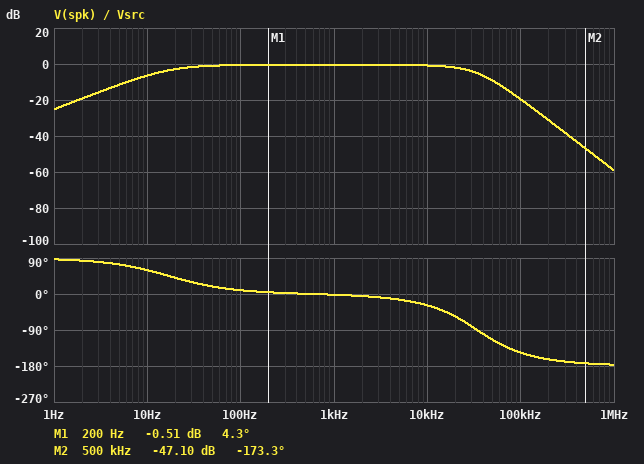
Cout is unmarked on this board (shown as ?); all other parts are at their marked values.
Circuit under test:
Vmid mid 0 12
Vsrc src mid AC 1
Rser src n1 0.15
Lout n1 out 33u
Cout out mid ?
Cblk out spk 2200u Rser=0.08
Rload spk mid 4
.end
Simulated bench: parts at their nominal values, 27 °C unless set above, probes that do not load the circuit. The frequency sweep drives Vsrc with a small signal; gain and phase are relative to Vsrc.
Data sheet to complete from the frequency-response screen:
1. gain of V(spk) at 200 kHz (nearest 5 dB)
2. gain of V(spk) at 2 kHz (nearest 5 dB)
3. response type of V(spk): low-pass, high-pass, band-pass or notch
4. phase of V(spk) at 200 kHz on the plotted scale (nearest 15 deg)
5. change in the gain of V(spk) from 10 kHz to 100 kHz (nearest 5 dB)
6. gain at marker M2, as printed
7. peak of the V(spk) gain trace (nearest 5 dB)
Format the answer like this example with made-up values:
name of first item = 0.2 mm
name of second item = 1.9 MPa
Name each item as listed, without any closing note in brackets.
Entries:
gain of V(spk) at 200 kHz = -30 dB
gain of V(spk) at 2 kHz = 0 dB
response type of V(spk): low-pass, high-pass, band-pass or notch = band-pass
phase of V(spk) at 200 kHz on the plotted scale = -165 deg
change in the gain of V(spk) from 10 kHz to 100 kHz = -20 dB
gain at marker M2, as printed = -47.10 dB
peak of the V(spk) gain trace = 0 dB
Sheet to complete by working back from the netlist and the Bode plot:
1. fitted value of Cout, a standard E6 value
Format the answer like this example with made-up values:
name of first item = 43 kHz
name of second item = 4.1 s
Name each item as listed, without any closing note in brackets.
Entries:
fitted value of Cout, a standard E6 value = 680 nF
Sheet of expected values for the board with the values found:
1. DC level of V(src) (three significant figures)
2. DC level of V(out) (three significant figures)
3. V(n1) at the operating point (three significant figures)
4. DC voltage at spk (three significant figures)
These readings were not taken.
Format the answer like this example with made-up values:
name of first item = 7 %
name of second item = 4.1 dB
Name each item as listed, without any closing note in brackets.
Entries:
DC level of V(src) = 12.0 V
DC level of V(out) = 12.0 V
V(n1) at the operating point = 12.0 V
DC voltage at spk = 12.0 V
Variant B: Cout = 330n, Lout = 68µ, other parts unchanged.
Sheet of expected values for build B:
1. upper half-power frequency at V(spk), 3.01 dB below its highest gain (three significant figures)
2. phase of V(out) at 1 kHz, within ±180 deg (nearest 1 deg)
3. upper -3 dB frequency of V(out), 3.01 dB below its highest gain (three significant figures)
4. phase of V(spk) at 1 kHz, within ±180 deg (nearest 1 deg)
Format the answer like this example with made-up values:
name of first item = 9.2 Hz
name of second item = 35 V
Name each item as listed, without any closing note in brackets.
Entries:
upper half-power frequency at V(spk), 3.01 dB below its highest gain = 10.8 kHz
phase of V(out) at 1 kHz, within ±180 deg = -6 deg
upper -3 dB frequency of V(out), 3.01 dB below its highest gain = 10.0 kHz
phase of V(spk) at 1 kHz, within ±180 deg = -5 deg
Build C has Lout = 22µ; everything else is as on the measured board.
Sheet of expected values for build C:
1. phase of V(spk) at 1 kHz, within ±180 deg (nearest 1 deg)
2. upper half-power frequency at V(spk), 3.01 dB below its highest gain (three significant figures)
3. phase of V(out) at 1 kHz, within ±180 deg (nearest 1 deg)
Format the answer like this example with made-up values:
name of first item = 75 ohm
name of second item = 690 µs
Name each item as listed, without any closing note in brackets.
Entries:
phase of V(spk) at 1 kHz, within ±180 deg = -1 deg
upper half-power frequency at V(spk), 3.01 dB below its highest gain = 42.4 kHz
phase of V(out) at 1 kHz, within ±180 deg = -2 deg
